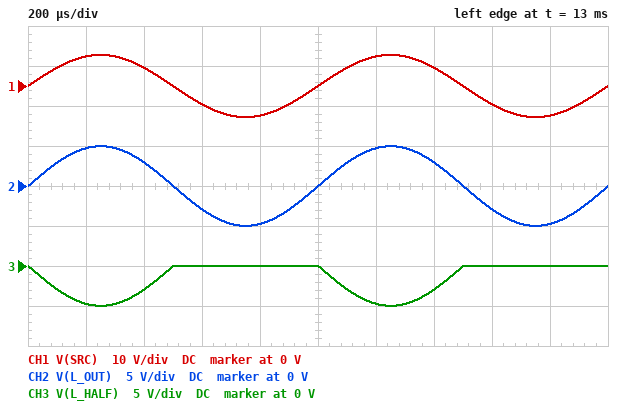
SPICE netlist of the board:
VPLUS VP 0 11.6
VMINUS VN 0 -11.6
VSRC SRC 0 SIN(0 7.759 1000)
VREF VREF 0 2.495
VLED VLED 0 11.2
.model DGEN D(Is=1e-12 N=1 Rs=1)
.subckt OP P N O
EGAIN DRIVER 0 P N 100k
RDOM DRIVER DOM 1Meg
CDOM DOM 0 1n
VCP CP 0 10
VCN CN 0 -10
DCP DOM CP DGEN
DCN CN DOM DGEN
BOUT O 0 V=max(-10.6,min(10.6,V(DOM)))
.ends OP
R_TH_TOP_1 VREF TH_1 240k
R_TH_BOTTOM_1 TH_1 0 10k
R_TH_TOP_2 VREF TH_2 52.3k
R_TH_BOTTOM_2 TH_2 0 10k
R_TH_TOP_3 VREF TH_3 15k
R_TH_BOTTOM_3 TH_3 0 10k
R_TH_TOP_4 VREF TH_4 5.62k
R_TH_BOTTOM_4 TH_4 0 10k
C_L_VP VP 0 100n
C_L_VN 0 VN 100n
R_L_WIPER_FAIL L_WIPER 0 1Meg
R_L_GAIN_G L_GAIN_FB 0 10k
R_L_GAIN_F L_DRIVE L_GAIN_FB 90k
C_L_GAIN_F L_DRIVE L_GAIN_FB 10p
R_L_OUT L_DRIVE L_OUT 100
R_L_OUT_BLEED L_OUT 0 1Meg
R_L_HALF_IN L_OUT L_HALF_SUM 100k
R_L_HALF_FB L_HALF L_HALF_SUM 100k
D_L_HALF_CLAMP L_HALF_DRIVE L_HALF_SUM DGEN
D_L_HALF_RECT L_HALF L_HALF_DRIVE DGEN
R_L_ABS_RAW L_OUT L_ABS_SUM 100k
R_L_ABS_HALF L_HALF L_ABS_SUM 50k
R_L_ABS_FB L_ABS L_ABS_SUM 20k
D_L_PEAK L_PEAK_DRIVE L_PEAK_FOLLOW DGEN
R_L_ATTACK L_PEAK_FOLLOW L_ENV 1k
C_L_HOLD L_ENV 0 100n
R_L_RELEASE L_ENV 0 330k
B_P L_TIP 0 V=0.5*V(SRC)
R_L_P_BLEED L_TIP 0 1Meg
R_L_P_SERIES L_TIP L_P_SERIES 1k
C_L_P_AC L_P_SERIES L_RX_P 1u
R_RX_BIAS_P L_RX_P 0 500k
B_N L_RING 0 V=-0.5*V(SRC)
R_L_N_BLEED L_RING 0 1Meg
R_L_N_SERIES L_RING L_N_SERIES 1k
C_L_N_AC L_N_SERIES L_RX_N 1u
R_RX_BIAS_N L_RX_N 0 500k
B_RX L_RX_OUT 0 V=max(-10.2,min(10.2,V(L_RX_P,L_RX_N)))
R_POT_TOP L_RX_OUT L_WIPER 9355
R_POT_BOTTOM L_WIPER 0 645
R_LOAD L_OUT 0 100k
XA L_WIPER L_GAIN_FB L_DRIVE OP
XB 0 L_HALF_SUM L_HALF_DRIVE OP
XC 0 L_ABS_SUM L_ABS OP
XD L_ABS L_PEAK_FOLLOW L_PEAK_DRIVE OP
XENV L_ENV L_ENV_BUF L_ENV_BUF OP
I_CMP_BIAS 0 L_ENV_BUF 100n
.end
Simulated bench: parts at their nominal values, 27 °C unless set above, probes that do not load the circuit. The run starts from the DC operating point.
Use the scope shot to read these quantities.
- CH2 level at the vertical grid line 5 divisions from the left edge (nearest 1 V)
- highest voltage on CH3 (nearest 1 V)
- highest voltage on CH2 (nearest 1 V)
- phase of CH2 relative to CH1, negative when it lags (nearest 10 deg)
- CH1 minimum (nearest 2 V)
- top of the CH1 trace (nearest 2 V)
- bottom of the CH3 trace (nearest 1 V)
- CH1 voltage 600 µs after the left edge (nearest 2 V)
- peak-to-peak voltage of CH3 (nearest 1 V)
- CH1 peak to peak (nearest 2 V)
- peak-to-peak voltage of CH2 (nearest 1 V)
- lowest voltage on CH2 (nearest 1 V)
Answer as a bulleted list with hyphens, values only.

- 0 V
- 0 V
- 5 V
- 0 deg
- -8 V
- 8 V
- -5 V
- -4 V
- 5 V
- 16 V
- 10 V
- -5 V
